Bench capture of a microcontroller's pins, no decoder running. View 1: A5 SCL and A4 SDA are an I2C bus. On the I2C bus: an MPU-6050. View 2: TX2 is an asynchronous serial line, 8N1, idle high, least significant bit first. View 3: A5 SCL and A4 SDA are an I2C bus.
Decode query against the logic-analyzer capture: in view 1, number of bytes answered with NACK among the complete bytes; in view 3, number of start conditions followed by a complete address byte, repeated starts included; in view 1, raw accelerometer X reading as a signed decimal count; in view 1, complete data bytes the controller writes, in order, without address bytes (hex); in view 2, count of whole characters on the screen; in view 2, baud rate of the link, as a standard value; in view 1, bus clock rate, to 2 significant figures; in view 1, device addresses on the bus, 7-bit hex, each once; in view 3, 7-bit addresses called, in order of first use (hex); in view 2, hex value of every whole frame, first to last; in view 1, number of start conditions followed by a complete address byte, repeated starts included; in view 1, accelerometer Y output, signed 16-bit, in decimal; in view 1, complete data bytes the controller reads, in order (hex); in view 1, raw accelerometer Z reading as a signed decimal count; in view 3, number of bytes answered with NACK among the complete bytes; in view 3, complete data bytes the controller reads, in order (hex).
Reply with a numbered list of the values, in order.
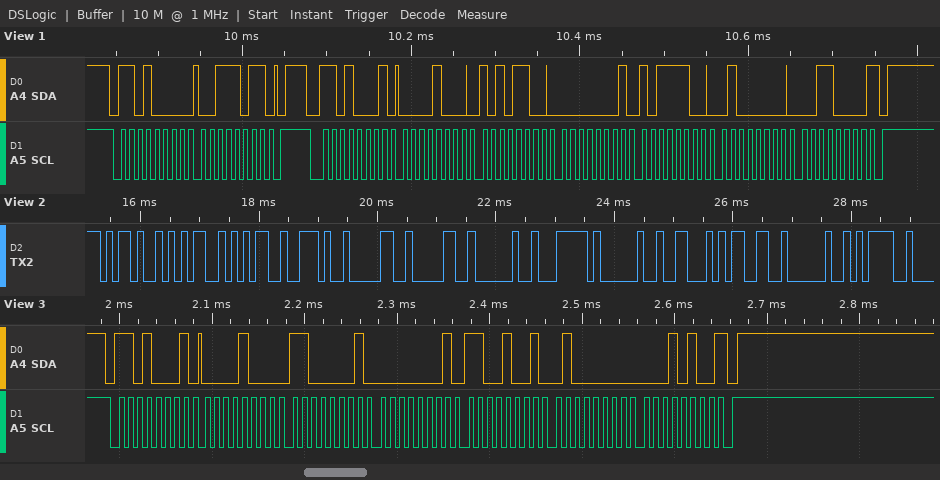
1. 1
2. 1
3. 2220
4. 3B
5. 13
6. 9600 baud
7. 100 kHz
8. 0x68
9. 0x68
10. 2D 35 35 2E 30 30 20 7C 20 46 33 20 3D
11. 2
12. 444
13. 08 AC 01 BC 40 30
14. 16432
15. 1
16. 08 C1 01 C9 40 14
